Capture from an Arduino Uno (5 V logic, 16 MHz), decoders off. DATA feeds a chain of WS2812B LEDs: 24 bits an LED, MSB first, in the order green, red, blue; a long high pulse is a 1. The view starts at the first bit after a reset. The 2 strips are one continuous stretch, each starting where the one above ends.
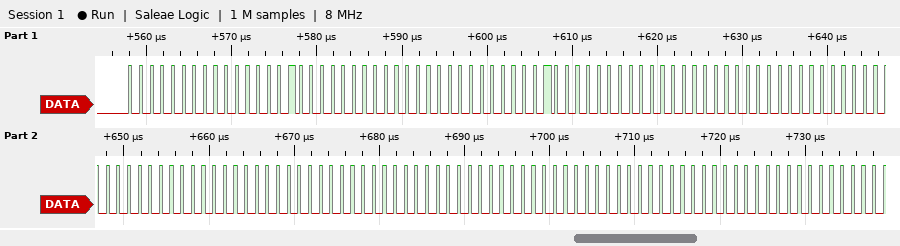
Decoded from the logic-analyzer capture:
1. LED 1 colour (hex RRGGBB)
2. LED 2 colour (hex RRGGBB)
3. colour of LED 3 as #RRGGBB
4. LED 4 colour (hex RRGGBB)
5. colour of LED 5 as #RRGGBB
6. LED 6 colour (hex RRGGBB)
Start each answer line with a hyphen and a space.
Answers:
- #010000
- #010000
- #000000
- #000000
- #000000
- #000000
